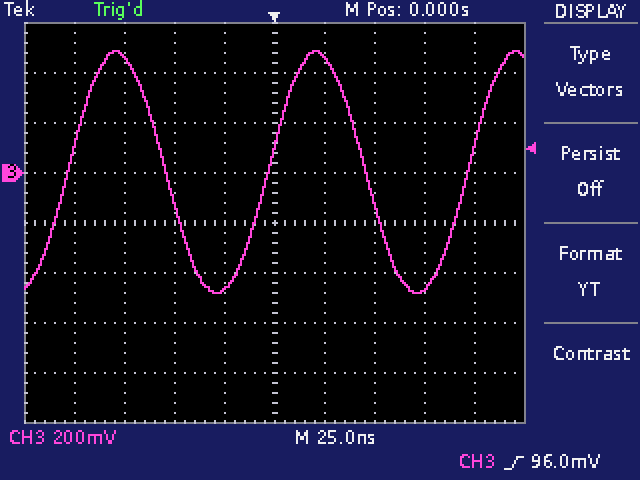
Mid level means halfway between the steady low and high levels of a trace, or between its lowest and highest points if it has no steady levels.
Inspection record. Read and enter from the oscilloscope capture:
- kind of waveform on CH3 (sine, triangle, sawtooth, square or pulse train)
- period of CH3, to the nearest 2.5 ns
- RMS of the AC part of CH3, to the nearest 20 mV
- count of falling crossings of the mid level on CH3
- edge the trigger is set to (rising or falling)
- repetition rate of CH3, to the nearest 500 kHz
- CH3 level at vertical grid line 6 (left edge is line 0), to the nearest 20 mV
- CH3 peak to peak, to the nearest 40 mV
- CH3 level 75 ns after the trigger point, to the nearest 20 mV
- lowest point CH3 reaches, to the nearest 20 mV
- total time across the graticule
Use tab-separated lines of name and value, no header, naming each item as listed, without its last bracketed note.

kind of waveform on CH3	sine
period of CH3, to the nearest 2.5 ns	100.0 ns
RMS of the AC part of CH3, to the nearest 20 mV	340 mV
count of falling crossings of the mid level on CH3	2
edge the trigger is set to	rising
repetition rate of CH3, to the nearest 500 kHz	10.0 MHz
CH3 level at vertical grid line 6 (left edge is line 0), to the nearest 20 mV	460 mV
CH3 peak to peak, to the nearest 40 mV	960 mV
CH3 level 75 ns after the trigger point, to the nearest 20 mV	-460 mV
lowest point CH3 reaches, to the nearest 20 mV	-480 mV
total time across the graticule	250 ns
